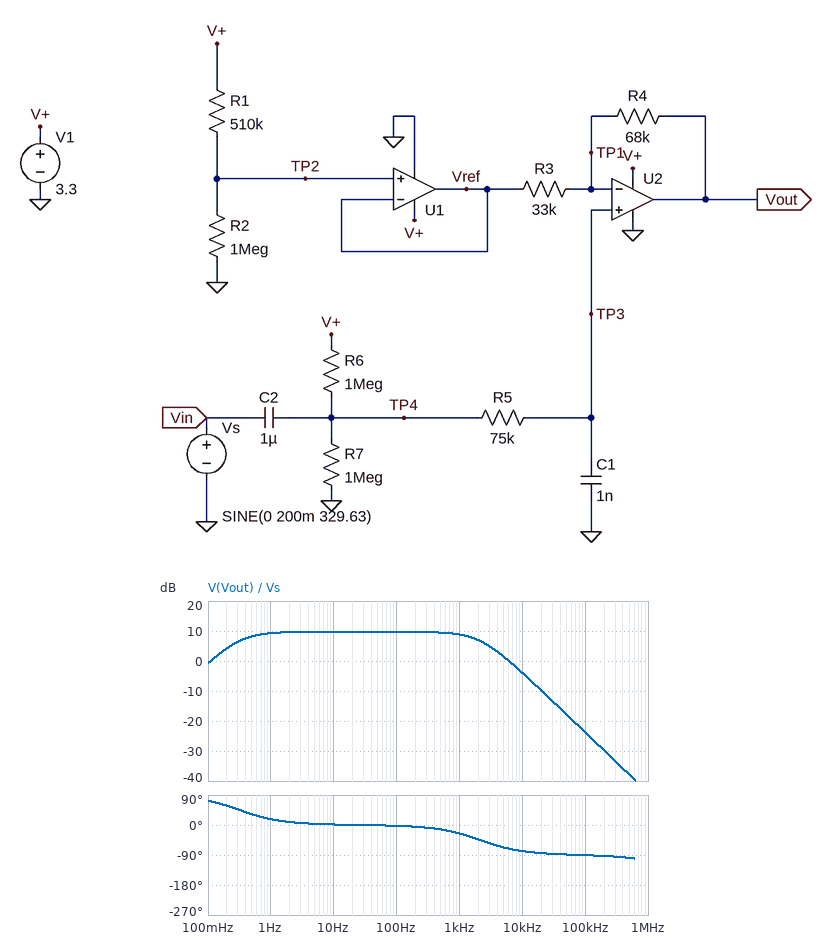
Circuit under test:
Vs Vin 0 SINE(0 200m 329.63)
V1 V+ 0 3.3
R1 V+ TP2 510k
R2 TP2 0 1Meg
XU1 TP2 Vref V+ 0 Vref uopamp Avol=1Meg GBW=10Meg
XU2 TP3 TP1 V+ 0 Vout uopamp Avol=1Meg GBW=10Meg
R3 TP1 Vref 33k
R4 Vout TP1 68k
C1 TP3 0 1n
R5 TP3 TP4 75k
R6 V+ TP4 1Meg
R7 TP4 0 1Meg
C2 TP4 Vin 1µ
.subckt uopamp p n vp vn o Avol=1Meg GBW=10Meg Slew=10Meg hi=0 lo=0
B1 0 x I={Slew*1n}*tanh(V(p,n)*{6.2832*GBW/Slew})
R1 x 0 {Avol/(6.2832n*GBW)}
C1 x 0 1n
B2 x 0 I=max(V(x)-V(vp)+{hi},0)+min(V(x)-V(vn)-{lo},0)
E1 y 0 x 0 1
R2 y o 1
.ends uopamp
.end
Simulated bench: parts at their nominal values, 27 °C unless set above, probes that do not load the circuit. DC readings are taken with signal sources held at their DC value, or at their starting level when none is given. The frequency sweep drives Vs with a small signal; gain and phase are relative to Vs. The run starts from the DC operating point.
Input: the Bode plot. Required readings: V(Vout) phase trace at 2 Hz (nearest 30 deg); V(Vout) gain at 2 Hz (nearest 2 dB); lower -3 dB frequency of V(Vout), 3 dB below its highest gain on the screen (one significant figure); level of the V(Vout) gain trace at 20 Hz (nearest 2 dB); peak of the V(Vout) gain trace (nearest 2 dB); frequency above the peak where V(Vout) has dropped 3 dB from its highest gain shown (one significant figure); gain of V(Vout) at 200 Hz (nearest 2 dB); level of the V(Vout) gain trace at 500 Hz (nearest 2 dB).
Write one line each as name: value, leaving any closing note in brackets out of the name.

V(Vout) phase trace at 2 Hz: 0 deg
V(Vout) gain at 2 Hz: 10 dB
lower -3 dB frequency of V(Vout), 3 dB below its highest gain on the screen: 300 mHz
level of the V(Vout) gain trace at 20 Hz: 10 dB
peak of the V(Vout) gain trace: 10 dB
frequency above the peak where V(Vout) has dropped 3 dB from its highest gain shown: 2 kHz
gain of V(Vout) at 200 Hz: 10 dB
level of the V(Vout) gain trace at 500 Hz: 10 dB
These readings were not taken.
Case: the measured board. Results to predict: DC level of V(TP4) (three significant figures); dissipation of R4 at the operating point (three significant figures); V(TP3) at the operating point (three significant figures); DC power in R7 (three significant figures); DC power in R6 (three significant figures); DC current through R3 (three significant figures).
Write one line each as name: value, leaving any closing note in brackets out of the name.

DC level of V(TP4): 1.65 V
dissipation of R4 at the operating point: 17.9 µW
V(TP3) at the operating point: 1.65 V
DC power in R7: 2.72 µW
DC power in R6: 2.72 µW
DC current through R3: 16.2 µA
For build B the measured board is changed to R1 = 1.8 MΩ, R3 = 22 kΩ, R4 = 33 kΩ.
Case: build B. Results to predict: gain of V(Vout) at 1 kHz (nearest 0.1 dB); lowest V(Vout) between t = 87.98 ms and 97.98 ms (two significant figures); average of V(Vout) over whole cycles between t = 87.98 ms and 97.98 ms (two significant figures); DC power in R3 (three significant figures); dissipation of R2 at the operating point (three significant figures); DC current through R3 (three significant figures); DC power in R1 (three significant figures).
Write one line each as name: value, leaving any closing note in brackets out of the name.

gain of V(Vout) at 1 kHz: 7.1 dB
lowest V(Vout) between t = 87.98 ms and 97.98 ms: 1.9 V
average of V(Vout) over whole cycles between t = 87.98 ms and 97.98 ms: 2.4 V
DC power in R3: 10.1 µW
dissipation of R2 at the operating point: 1.39 µW
DC current through R3: 21.4 µA
DC power in R1: 2.50 µW
